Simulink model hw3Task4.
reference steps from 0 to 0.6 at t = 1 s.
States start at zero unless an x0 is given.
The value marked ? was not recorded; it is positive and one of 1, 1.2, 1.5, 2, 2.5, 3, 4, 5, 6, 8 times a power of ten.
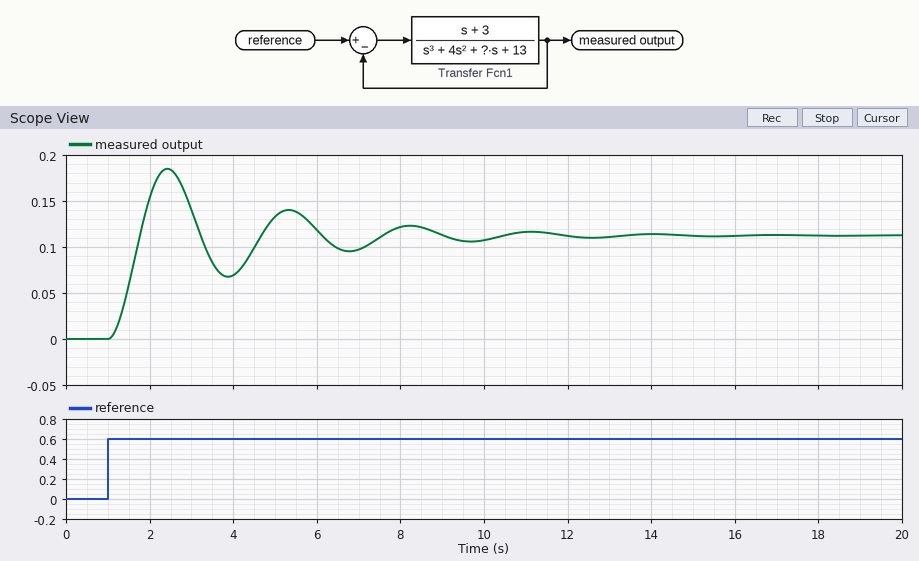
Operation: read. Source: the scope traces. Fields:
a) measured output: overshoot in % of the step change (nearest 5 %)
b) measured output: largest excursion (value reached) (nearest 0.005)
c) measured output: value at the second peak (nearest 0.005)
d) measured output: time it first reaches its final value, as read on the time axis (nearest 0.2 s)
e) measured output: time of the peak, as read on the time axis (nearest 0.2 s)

65 %
0.185
0.140
1.8 s
2.4 s
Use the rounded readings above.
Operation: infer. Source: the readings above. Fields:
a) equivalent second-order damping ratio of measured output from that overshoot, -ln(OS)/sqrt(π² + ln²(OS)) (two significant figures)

0.14
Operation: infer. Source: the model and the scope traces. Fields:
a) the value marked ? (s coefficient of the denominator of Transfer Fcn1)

6
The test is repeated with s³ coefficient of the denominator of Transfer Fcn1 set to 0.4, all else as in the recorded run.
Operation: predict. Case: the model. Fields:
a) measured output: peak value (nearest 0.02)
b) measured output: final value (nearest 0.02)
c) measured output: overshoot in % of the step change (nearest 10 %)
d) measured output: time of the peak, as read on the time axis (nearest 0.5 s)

0.16
0.12
40 %
2.5 s
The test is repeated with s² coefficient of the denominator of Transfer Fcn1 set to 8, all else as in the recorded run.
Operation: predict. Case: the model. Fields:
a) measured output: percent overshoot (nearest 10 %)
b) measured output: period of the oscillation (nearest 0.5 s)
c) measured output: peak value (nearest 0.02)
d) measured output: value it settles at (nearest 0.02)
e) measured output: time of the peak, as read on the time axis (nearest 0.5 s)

50 %
4.5 s
0.18
0.12
3.0 s
